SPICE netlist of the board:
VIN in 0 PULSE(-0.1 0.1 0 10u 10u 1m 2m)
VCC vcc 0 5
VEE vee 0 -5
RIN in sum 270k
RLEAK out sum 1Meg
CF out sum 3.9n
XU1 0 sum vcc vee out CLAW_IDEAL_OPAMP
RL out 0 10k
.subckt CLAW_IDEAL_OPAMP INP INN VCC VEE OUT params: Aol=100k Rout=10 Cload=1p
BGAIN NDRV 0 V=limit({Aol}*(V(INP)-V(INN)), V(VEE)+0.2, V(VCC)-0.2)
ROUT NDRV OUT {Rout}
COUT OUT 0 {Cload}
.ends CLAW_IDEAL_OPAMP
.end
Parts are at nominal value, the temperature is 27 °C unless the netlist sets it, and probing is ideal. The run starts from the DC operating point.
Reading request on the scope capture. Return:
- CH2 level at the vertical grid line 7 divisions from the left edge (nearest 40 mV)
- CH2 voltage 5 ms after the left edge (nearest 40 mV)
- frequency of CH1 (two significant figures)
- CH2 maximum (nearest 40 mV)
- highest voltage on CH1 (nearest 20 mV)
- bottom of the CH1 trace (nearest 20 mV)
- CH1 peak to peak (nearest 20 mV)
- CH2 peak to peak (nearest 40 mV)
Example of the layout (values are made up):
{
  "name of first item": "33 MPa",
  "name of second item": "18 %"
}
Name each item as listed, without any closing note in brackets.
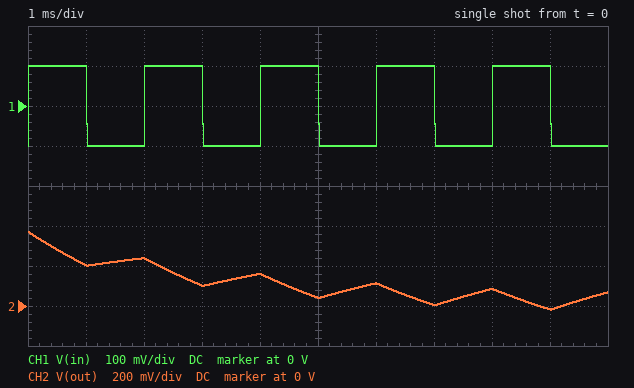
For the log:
{
  "CH2 level at the vertical grid line 7 divisions from the left edge": "0 V",
  "CH2 voltage 5 ms after the left edge": "40 mV",
  "frequency of CH1": "500 Hz",
  "CH2 maximum": "360 mV",
  "highest voltage on CH1": "100 mV",
  "bottom of the CH1 trace": "-100 mV",
  "CH1 peak to peak": "200 mV",
  "CH2 peak to peak": "400 mV"
}
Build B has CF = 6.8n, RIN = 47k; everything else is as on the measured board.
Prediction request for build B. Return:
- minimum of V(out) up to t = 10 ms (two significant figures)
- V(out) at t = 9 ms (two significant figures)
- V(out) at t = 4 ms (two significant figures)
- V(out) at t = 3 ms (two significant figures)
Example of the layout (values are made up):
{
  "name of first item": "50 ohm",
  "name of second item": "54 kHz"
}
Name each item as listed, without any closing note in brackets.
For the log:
{
  "minimum of V(out) up to t = 10 ms": "350 mV",
  "V(out) at t = 9 ms": "360 mV",
  "V(out) at t = 4 ms": "1.2 V",
  "V(out) at t = 3 ms": "1.1 V"
}
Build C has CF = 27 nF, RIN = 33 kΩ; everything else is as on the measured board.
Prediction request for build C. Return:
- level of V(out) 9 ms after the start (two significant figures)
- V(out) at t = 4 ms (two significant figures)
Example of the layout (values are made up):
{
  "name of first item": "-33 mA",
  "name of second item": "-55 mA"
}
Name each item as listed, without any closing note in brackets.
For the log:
{
  "level of V(out) 9 ms after the start": "2.1 V",
  "V(out) at t = 4 ms": "2.6 V"
}
